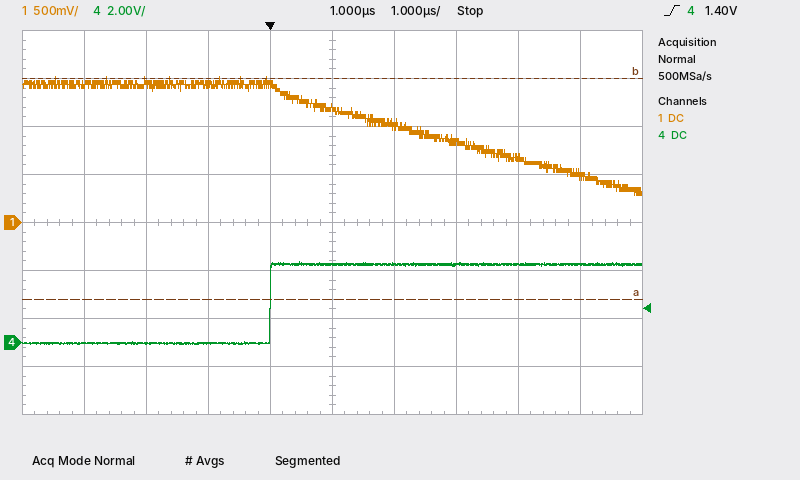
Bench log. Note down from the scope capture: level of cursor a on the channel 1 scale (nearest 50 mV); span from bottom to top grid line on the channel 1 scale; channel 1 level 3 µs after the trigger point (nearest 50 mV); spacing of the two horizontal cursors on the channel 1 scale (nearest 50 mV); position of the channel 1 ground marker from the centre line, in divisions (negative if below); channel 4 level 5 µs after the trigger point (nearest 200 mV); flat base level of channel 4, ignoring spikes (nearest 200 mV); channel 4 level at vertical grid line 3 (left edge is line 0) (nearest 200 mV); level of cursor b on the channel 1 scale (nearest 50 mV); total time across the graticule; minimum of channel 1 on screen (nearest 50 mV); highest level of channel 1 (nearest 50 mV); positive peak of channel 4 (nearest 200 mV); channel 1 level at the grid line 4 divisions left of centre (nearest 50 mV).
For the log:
-800 mV
4 V
850 mV
2.30 V
0.0 div
3.2 V
0.0 V
0.0 V
1.50 V
10 µs
300 mV
1.50 V
3.4 V
1.45 V
